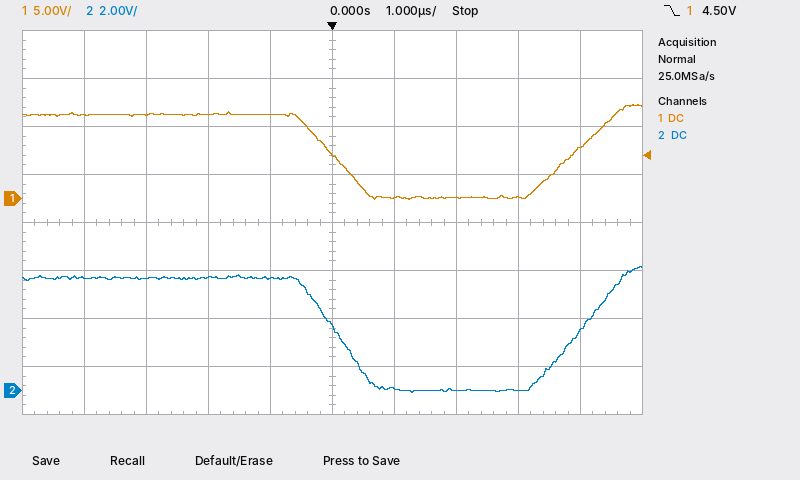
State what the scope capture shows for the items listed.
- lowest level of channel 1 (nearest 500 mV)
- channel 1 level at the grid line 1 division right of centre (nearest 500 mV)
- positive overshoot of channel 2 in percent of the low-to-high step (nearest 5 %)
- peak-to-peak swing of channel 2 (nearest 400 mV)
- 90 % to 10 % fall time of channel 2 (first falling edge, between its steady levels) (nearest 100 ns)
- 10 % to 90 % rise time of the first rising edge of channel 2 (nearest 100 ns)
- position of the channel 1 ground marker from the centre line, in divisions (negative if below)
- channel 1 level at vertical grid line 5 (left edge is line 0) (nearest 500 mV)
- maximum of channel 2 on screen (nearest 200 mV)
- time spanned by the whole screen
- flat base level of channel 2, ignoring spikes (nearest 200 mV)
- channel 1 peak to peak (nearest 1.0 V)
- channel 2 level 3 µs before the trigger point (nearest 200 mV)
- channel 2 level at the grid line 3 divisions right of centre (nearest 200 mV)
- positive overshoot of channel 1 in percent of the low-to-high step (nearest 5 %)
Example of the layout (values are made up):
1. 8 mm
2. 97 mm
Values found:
1. 0.0 V
2. 0.0 V
3. 10 %
4. 5.2 V
5. 1.0 µs
6. 1.2 µs
7. +0.5 div
8. 4.5 V
9. 5.2 V
10. 10 µs
11. 0.0 V
12. 10.0 V
13. 4.6 V
14. 0.0 V
15. 10 %
